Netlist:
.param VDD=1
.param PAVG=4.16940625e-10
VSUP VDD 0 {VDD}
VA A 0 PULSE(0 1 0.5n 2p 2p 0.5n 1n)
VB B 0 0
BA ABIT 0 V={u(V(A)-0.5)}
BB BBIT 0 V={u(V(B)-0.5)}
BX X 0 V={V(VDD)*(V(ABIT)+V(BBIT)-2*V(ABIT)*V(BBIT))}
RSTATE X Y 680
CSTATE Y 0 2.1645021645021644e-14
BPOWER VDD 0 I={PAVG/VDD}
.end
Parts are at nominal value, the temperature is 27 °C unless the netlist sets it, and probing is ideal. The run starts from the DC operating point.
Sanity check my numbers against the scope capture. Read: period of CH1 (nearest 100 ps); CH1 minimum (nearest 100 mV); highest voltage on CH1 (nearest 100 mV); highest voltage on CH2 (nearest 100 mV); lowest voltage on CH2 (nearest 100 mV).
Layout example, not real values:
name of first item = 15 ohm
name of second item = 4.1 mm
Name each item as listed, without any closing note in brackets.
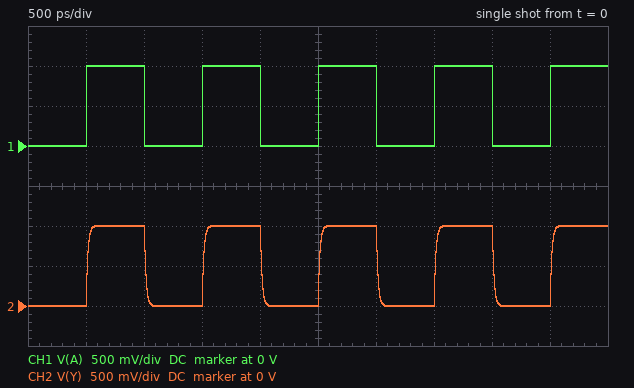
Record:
period of CH1 = 1.0 ns
CH1 minimum = 0 V
highest voltage on CH1 = 1.0 V
highest voltage on CH2 = 1.0 V
lowest voltage on CH2 = 0 V
